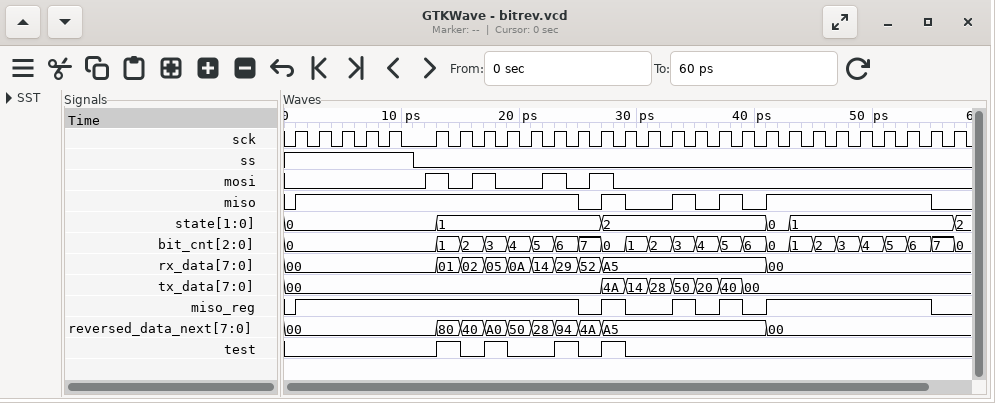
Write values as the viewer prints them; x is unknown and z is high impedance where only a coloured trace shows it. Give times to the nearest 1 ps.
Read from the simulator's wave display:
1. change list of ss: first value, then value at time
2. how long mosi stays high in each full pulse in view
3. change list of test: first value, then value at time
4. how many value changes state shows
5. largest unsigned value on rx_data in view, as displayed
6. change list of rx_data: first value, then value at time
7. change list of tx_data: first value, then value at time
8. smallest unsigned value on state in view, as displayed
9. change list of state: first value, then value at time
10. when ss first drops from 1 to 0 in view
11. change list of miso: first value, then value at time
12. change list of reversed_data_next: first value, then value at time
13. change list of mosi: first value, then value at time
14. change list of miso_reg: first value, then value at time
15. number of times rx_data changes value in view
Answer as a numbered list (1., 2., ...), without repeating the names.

1. 1, 0 at 11 ps
2. 2 ps, 2 ps, 2 ps, 2 ps
3. 0, 1 at 13 ps, 0 at 15 ps, 1 at 17 ps, 0 at 19 ps, 1 at 23 ps, 0 at 25 ps, 1 at 27 ps, 0 at 29 ps
4. 5
5. A5
6. 00, 01 at 13 ps, 02 at 15 ps, 05 at 17 ps, 0A at 19 ps, 14 at 21 ps, 29 at 23 ps, 52 at 25 ps, A5 at 27 ps, 00 at 41 ps
7. 00, 4A at 27 ps, 14 at 29 ps, 28 at 31 ps, 50 at 33 ps, 20 at 35 ps, 40 at 37 ps, 00 at 39 ps
8. 0
9. 0, 1 at 13 ps, 2 at 27 ps, 0 at 41 ps, 1 at 43 ps, 2 at 57 ps
10. 11 ps
11. 0, 1 at 1 ps, 0 at 25 ps, 1 at 27 ps, 0 at 29 ps, 1 at 33 ps, 0 at 35 ps, 1 at 37 ps, 0 at 39 ps, 1 at 41 ps, 0 at 55 ps
12. 00, 80 at 13 ps, 40 at 15 ps, A0 at 17 ps, 50 at 19 ps, 28 at 21 ps, 94 at 23 ps, 4A at 25 ps, A5 at 27 ps, 00 at 41 ps
13. 0, 1 at 12 ps, 0 at 14 ps, 1 at 16 ps, 0 at 18 ps, 1 at 22 ps, 0 at 24 ps, 1 at 26 ps, 0 at 28 ps
14. 0, 1 at 1 ps, 0 at 25 ps, 1 at 27 ps, 0 at 29 ps, 1 at 33 ps, 0 at 35 ps, 1 at 37 ps, 0 at 39 ps, 1 at 41 ps, 0 at 55 ps
15. 9
